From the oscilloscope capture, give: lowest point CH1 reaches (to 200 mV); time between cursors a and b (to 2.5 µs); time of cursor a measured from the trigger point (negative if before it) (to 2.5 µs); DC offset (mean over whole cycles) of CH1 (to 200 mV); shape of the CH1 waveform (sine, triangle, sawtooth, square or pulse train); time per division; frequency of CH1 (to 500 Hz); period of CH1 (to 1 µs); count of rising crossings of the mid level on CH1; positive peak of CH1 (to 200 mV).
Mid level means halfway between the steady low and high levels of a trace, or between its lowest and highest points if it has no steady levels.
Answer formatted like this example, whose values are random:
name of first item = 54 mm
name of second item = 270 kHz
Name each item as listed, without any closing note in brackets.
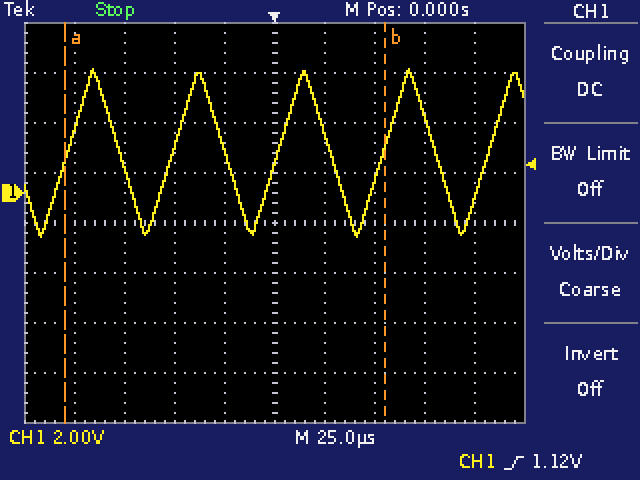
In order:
lowest point CH1 reaches = -1.8 V
time between cursors a and b = 160.0 µs
time of cursor a measured from the trigger point (negative if before it) = -105.0 µs
DC offset (mean over whole cycles) of CH1 = 1.6 V
shape of the CH1 waveform = triangle
time per division = 25 µs
frequency of CH1 = 19.0 kHz
period of CH1 = 53 µs
count of rising crossings of the mid level on CH1 = 5
positive peak of CH1 = 5.0 V
